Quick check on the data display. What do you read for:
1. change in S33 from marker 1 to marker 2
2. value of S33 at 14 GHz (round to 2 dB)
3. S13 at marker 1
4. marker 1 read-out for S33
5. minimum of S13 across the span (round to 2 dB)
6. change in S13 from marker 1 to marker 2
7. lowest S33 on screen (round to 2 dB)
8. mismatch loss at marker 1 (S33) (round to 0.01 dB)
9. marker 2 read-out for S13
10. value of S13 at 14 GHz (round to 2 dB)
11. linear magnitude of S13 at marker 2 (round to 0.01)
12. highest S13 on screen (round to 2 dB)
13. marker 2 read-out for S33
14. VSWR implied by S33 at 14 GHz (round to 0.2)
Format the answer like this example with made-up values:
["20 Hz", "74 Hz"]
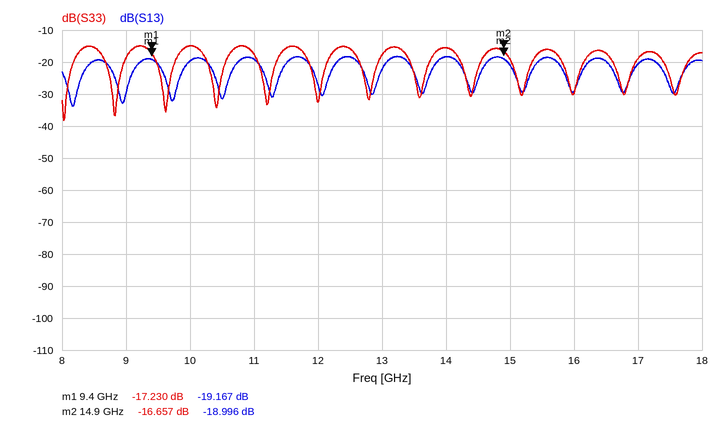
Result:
["0.573 dB", "-16 dB", "-19.167 dB", "-17.230 dB", "-34 dB", "0.171 dB", "-38 dB", "0.08 dB", "-18.996 dB", "-18 dB", "0.11", "-18 dB", "-16.657 dB", "1.4"]
